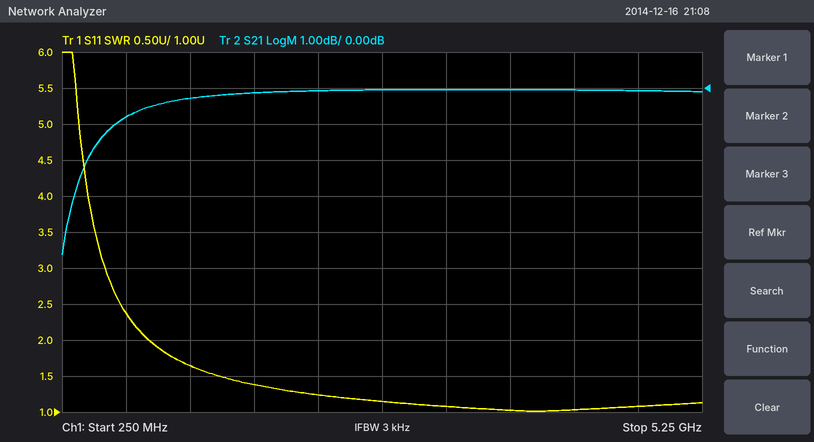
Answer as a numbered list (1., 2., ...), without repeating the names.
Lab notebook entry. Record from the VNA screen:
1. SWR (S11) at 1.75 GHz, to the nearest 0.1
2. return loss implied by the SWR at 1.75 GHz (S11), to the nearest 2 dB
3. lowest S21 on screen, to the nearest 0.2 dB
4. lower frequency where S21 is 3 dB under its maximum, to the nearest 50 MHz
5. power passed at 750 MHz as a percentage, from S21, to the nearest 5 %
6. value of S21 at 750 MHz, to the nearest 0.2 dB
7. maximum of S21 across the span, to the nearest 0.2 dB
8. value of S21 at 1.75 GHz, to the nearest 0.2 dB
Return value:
1. 1.4
2. 16 dB
3. -4.6 dB
4. 350 MHz
5. 85 %
6. -0.8 dB
7. 0.0 dB
8. -0.2 dB
